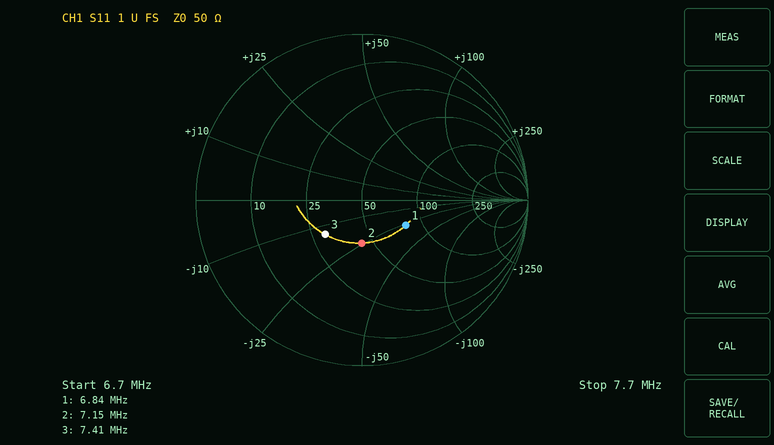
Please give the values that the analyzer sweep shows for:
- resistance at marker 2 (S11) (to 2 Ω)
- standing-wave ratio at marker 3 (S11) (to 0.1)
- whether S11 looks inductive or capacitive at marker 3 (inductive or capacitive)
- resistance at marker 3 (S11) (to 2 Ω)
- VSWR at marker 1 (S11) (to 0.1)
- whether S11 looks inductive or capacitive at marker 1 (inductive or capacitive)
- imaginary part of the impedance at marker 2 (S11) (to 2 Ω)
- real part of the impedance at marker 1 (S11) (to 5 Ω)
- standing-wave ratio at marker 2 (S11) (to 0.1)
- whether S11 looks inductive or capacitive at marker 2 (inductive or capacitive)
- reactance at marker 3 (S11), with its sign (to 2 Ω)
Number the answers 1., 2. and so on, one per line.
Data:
1. 44 Ω
2. 1.9
3. capacitive
4. 30 Ω
5. 1.9
6. capacitive
7. -24 Ω
8. 80 Ω
9. 1.7
10. capacitive
11. -14 Ω
